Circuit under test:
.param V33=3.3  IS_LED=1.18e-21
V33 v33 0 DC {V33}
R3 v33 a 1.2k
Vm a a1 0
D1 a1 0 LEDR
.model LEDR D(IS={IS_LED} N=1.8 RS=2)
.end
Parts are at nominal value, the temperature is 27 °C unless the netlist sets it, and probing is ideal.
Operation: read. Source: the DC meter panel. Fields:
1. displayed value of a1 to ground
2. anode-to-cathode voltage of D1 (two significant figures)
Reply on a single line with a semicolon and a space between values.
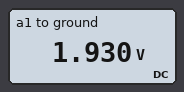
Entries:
1.930 V; 1.9 V
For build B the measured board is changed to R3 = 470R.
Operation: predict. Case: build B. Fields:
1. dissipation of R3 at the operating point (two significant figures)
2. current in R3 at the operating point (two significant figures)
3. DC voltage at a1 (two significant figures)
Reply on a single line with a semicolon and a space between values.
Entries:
3.7 mW; 2.8 mA; 2.0 V
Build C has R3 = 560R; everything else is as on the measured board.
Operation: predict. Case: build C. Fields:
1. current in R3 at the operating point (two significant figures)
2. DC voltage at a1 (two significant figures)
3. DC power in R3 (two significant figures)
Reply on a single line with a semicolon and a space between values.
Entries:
2.4 mA; 2.0 V; 3.2 mW
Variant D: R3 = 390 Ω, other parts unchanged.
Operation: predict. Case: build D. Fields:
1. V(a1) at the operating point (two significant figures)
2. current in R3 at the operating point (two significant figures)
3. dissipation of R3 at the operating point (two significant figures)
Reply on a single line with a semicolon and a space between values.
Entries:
2.0 V; 3.4 mA; 4.4 mW
